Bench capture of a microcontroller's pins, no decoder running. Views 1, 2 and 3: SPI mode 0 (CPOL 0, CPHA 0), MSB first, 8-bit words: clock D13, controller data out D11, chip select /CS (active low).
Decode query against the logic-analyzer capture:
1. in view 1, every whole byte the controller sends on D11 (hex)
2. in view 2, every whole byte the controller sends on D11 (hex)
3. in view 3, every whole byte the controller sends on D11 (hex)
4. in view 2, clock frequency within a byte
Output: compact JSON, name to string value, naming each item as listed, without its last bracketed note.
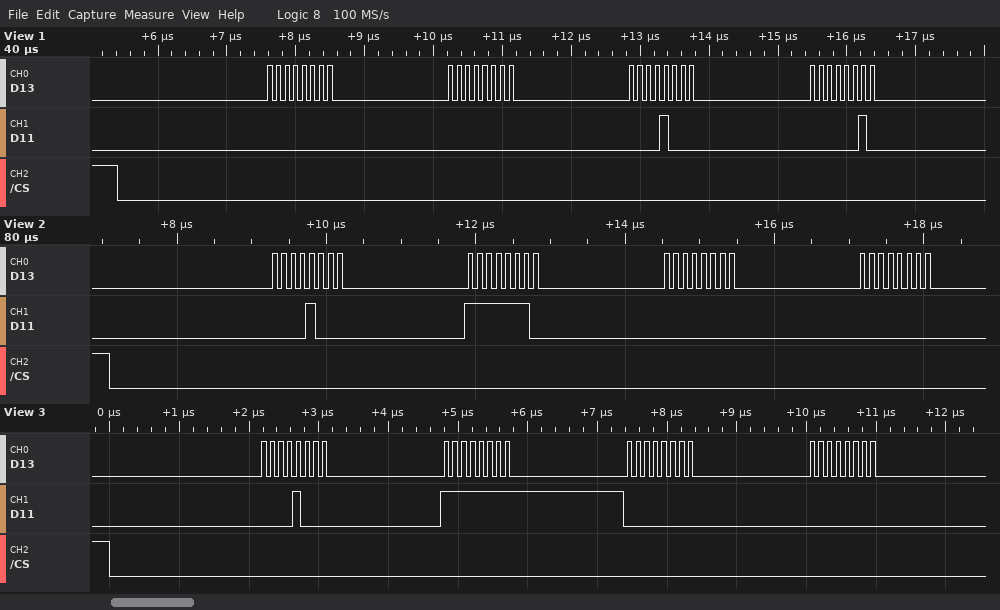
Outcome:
{"in view 1, every whole byte the controller sends on D11": "00 00 08 02", "in view 2, every whole byte the controller sends on D11": "0x08 0xFE 0x00 0x00", "in view 3, every whole byte the controller sends on D11": "08 FF 00 00", "in view 2, clock frequency within a byte": "8 MHz"}
